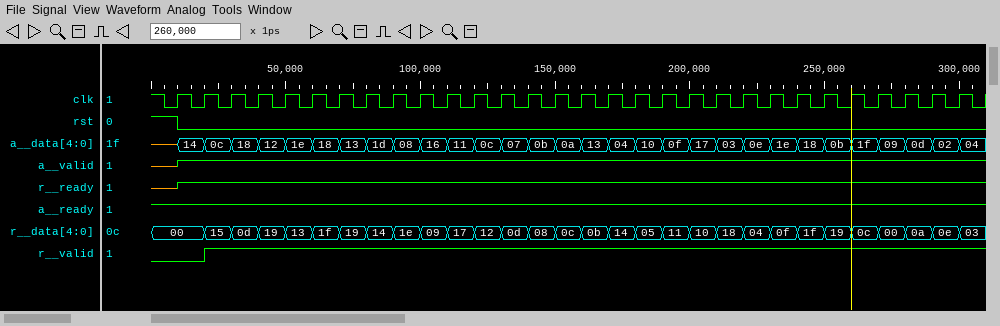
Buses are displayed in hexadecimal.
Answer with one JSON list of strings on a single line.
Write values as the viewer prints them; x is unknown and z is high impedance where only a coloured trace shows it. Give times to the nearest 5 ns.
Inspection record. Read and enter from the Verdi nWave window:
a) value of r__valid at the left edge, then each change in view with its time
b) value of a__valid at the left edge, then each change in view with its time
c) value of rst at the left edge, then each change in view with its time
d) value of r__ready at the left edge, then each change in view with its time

["0, 1 at 20 ns", "z, 1 at 10 ns", "1, 0 at 10 ns", "z, 1 at 10 ns"]
